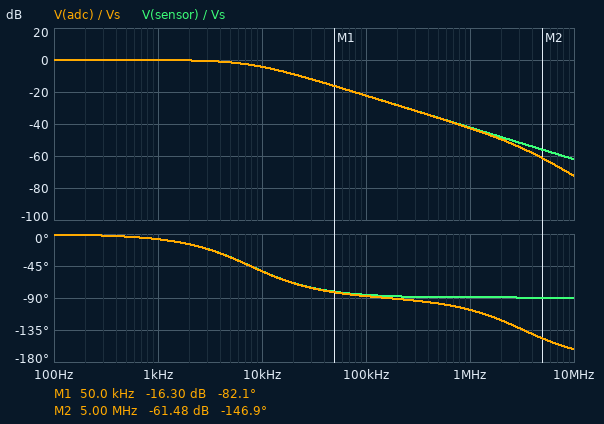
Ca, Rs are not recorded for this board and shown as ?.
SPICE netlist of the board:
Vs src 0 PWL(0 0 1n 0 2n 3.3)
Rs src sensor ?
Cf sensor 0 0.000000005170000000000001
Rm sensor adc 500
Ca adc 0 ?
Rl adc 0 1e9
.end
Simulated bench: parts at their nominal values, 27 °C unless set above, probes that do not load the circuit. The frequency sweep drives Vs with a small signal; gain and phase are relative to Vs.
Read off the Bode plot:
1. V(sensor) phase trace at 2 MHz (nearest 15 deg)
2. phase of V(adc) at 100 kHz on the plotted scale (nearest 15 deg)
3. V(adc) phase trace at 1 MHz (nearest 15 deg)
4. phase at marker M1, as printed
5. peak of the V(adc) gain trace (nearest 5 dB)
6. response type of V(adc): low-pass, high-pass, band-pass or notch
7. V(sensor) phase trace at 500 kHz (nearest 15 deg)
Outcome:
-90 deg
-90 deg
-105 deg
-82.1 deg
0 dB
low-pass
-90 deg
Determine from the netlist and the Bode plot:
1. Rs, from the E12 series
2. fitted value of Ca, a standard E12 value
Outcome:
3.9 kΩ
100 pF
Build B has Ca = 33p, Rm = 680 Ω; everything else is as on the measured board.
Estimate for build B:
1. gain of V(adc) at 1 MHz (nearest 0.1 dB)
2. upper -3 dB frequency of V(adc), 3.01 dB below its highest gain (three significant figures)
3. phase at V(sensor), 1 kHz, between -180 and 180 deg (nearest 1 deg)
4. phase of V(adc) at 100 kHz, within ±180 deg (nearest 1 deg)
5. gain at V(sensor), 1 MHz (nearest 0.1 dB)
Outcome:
-42.2 dB
7.84 kHz
-7 deg
-86 deg
-42.1 dB
